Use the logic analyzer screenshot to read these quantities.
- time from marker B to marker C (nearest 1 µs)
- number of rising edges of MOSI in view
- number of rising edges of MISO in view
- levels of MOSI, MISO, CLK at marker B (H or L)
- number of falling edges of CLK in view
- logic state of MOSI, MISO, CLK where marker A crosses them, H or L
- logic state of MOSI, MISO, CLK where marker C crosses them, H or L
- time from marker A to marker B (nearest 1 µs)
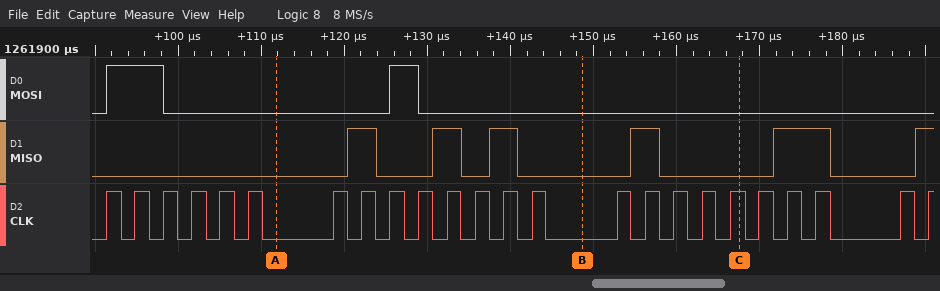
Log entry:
19 µs
2
6
MOSI=L, MISO=L, CLK=L
23
MOSI=L, MISO=L, CLK=L
MOSI=L, MISO=L, CLK=H
37 µs
